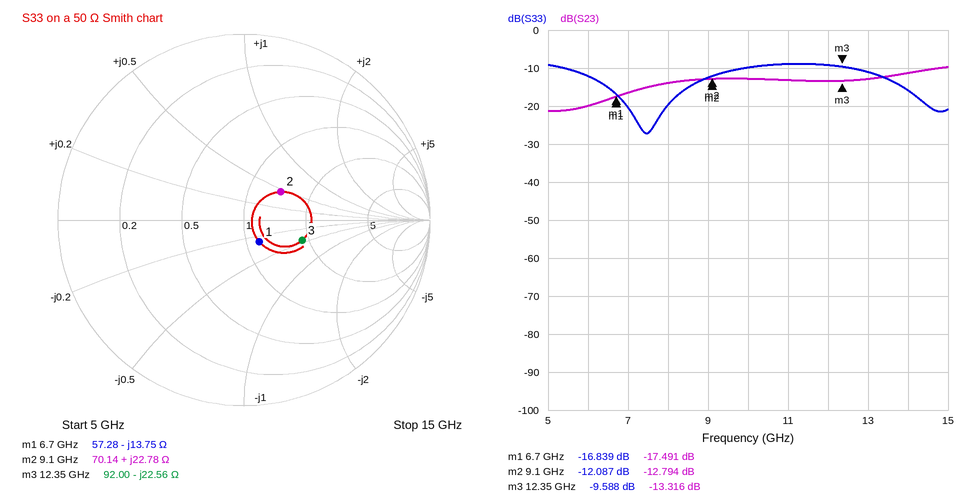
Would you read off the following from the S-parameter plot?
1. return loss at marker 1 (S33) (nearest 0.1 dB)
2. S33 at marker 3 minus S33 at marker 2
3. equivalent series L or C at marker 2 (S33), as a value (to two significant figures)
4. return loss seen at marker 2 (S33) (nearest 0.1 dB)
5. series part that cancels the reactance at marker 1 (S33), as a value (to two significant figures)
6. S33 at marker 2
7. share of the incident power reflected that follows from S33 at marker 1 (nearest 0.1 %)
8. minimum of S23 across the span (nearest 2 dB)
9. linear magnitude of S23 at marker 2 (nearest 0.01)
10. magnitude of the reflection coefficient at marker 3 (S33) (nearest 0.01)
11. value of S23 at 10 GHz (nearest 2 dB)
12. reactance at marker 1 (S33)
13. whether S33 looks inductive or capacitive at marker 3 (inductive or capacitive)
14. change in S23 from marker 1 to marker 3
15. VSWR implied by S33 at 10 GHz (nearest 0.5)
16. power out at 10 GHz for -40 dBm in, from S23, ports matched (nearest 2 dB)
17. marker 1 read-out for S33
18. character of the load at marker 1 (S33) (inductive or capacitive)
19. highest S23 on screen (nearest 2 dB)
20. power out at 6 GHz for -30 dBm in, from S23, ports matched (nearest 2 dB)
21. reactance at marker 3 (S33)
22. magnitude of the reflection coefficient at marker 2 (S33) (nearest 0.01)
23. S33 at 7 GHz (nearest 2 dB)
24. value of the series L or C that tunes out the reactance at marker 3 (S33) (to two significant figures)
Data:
16.8 dB
2.499 dB
400 pH
12.1 dB
330 pH
-12.087 dB
2.1 %
-22 dB
0.23
0.33
-12 dB
-13.75 Ω
capacitive
4.175 dB
2.0
-52 dBm
-16.839 dB
capacitive
-10 dB
-50 dBm
-22.56 Ω
0.25
-20 dB
290 pH
